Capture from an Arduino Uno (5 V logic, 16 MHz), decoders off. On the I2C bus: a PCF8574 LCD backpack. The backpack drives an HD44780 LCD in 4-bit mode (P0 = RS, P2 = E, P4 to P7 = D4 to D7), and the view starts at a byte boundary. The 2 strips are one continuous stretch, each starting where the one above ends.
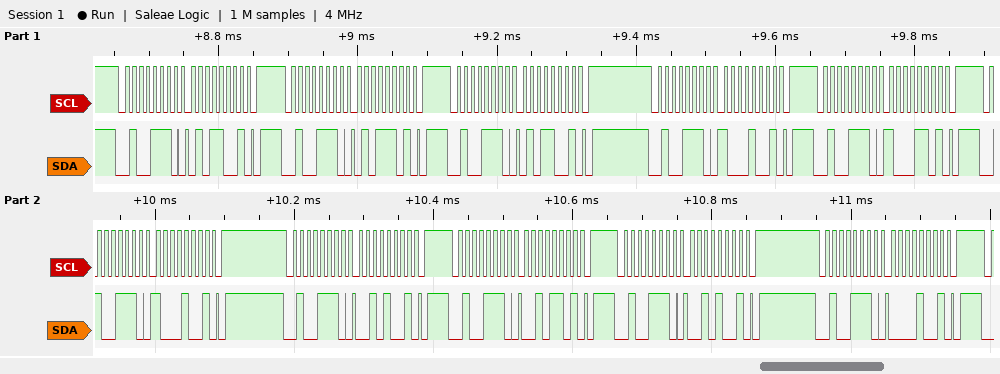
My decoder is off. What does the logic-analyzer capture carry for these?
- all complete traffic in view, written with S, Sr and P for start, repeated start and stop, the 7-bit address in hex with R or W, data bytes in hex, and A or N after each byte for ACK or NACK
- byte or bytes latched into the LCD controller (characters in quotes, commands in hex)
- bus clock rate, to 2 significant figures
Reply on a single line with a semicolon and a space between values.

S 27W A 59 A P S 27W A 5D A P S 27W A 59 A P S 27W A 89 A P S 27W A 8D A P S 27W A 89 A P S 27W A 29 A P S 27W A 2D A P S 27W A 29 A P S 27W A 09 A P; 'X'; 100 kHz
